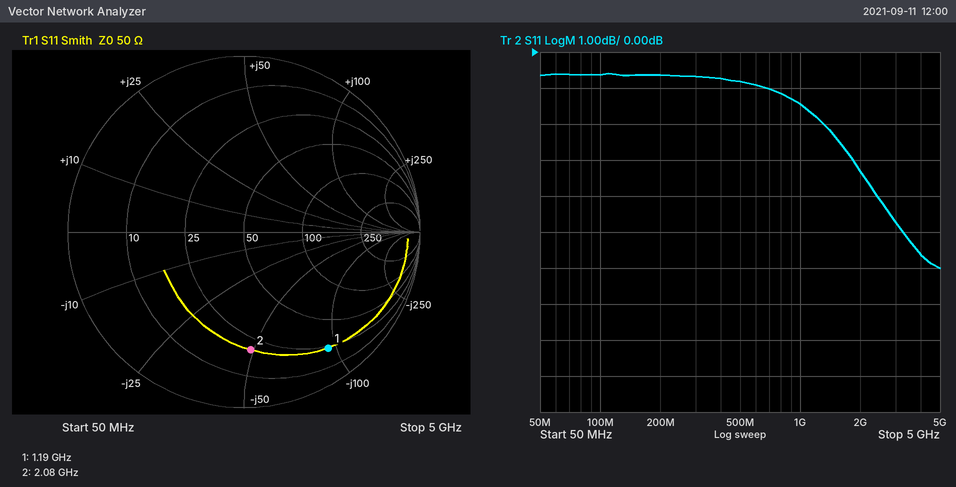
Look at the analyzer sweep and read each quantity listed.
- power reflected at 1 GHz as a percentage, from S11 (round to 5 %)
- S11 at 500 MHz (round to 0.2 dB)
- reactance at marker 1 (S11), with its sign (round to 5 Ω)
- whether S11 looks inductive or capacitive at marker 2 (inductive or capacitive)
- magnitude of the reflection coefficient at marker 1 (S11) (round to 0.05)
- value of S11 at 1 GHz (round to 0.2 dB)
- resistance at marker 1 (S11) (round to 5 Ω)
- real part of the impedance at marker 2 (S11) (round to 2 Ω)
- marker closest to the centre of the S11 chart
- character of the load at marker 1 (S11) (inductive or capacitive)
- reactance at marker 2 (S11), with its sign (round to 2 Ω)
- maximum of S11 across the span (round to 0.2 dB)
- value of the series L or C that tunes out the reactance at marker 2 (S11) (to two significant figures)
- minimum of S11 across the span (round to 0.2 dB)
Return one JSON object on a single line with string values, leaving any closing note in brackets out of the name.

{"power reflected at 1 GHz as a percentage, from S11": "70 %", "S11 at 500 MHz": "-0.8 dB", "reactance at marker 1 (S11), with its sign": "-95 Ω", "whether S11 looks inductive or capacitive at marker 2": "capacitive", "magnitude of the reflection coefficient at marker 1 (S11)": "0.80", "value of S11 at 1 GHz": "-1.4 dB", "resistance at marker 1 (S11)": "25 Ω", "real part of the impedance at marker 2 (S11)": "20 Ω", "marker closest to the centre of the S11 chart": "marker 2", "character of the load at marker 1 (S11)": "capacitive", "reactance at marker 2 (S11), with its sign": "-48 Ω", "maximum of S11 across the span": "-0.6 dB", "value of the series L or C that tunes out the reactance at marker 2 (S11)": "3.7 nH", "minimum of S11 across the span": "-6.0 dB"}
